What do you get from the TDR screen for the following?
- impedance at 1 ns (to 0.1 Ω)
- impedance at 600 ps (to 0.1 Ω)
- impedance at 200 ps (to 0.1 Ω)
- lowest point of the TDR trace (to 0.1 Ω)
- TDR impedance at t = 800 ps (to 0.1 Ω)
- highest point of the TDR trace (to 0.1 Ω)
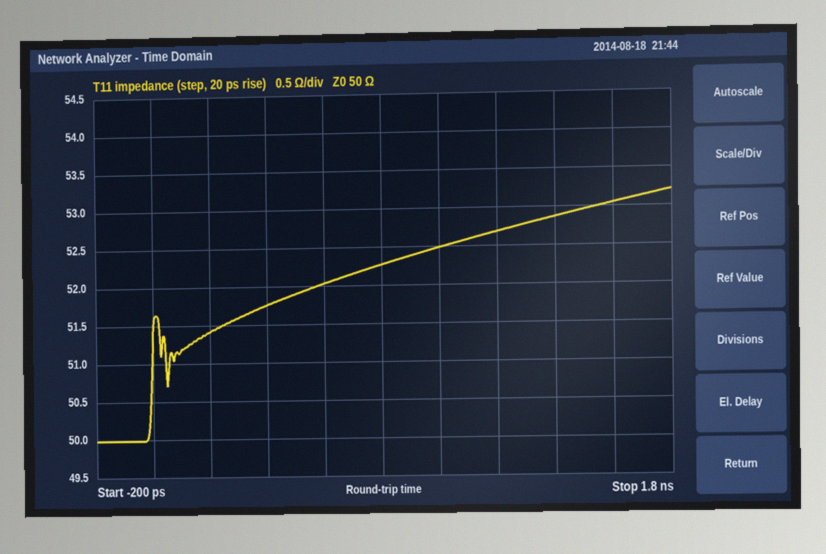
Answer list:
52.5 Ω
52.0 Ω
51.4 Ω
50.0 Ω
52.3 Ω
53.2 Ω
